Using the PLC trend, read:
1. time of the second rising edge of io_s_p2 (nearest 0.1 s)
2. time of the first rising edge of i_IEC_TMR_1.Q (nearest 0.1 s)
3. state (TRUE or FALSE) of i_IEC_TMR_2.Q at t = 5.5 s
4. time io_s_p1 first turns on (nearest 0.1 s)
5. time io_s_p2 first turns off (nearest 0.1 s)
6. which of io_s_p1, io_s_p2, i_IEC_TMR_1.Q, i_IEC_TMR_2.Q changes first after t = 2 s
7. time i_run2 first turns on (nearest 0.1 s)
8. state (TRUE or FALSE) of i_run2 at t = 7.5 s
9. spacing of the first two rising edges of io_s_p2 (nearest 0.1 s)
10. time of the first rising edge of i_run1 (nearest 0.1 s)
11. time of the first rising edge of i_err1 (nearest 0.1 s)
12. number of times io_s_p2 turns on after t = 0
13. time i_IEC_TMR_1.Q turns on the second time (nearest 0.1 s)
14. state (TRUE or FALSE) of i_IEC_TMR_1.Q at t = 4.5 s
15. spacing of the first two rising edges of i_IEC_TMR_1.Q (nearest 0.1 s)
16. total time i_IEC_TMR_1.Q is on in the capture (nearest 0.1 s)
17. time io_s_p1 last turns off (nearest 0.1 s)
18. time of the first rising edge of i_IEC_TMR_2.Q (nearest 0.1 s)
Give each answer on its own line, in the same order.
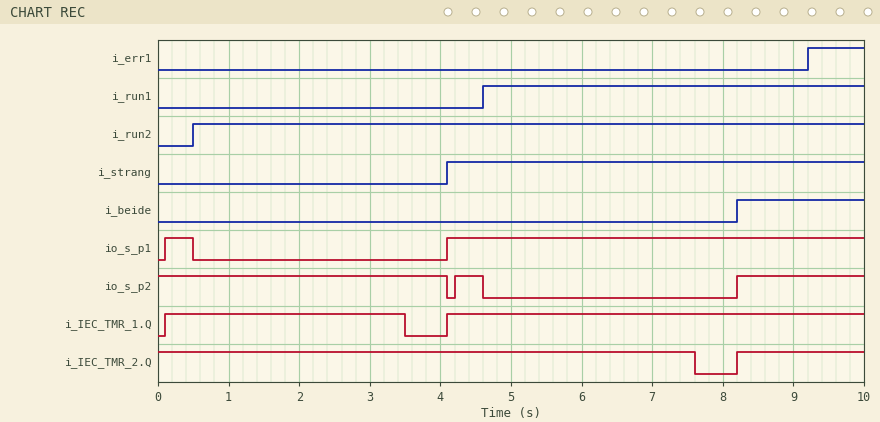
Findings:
8.2 s
0.1 s
TRUE
0.1 s
4.1 s
i_IEC_TMR_1.Q
0.5 s
TRUE
4.0 s
4.6 s
9.2 s
2
4.1 s
TRUE
4.0 s
9.3 s
0.5 s
8.2 s
